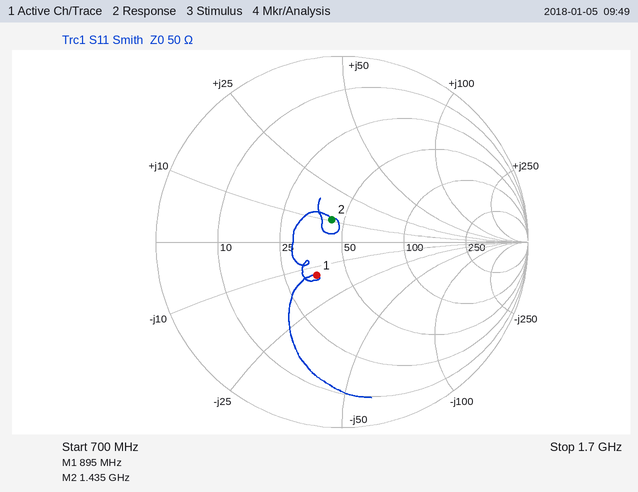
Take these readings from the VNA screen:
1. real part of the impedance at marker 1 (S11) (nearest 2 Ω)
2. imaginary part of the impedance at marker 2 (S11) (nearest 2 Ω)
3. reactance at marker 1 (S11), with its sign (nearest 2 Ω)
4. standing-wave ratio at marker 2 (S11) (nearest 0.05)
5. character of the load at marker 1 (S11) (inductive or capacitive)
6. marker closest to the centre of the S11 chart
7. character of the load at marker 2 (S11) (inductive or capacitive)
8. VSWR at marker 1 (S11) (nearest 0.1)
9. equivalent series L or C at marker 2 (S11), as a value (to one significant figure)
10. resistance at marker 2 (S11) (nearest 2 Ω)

36 Ω
+10 Ω
-14 Ω
1.30
capacitive
marker 2
inductive
1.6
1 nH
44 Ω
